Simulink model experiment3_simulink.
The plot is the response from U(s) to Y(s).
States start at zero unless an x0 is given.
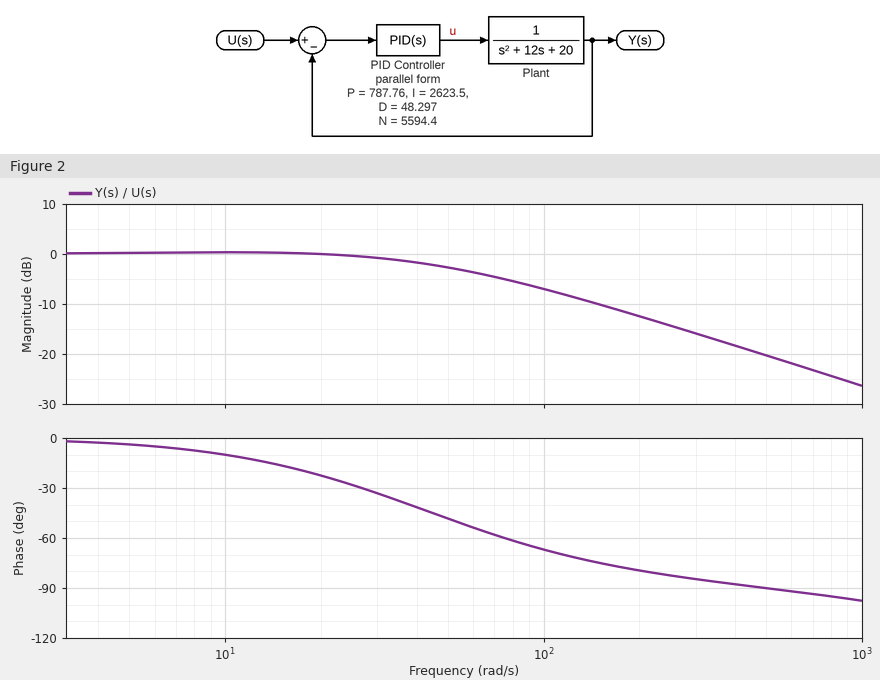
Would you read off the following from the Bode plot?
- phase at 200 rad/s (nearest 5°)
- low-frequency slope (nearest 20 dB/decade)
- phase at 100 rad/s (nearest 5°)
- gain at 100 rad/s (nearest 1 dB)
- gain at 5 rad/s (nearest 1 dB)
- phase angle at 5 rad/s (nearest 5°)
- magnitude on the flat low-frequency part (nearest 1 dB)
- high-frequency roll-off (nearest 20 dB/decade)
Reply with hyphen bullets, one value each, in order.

- -80°
- 0 dB/decade
- -65°
- -7 dB
- 0 dB
- -5°
- 0 dB
- -20 dB/decade
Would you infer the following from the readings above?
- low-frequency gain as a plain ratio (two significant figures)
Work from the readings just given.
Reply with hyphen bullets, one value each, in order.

- 1.0
